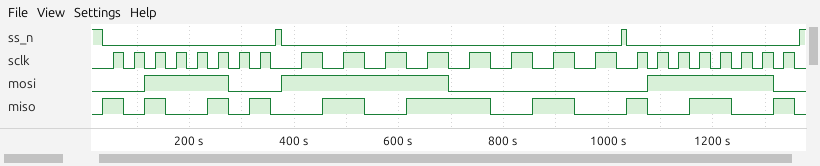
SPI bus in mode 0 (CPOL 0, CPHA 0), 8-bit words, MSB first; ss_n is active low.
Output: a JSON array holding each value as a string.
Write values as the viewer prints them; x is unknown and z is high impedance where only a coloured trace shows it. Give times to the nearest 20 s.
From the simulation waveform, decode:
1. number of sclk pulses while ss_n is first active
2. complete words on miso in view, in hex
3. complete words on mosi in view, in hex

["8", "A5, 5A, 99", "3C, F0, 7E"]
